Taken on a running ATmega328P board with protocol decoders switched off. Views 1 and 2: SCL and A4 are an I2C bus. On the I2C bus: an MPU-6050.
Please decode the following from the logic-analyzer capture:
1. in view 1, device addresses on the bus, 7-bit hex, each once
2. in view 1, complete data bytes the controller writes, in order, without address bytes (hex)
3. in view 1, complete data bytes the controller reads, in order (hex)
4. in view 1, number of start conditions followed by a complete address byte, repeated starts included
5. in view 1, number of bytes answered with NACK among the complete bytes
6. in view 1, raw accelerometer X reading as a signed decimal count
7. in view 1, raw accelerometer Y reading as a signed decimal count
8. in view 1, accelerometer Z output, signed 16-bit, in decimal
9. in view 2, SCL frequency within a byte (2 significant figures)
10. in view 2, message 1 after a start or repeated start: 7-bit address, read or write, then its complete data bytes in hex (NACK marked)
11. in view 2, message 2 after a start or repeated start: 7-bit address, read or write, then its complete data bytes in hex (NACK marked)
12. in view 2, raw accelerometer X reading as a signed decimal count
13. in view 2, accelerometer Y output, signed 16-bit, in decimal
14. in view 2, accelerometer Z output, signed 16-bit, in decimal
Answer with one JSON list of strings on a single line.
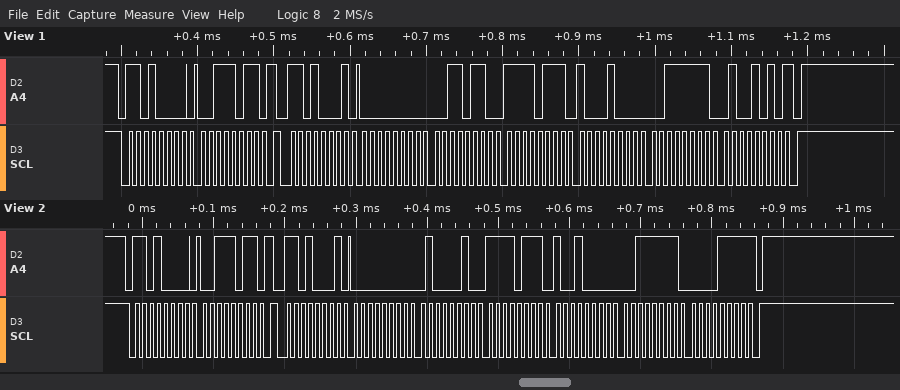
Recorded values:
["0x68", "3B", "00 36 F7 88 3F 4A", "2", "1", "54", "-2168", "16202", "100 kHz", "0x68 write: 3B", "0x68 read: 00 42 F7 90 3F 0F NACK", "66", "-2160", "16143"]
